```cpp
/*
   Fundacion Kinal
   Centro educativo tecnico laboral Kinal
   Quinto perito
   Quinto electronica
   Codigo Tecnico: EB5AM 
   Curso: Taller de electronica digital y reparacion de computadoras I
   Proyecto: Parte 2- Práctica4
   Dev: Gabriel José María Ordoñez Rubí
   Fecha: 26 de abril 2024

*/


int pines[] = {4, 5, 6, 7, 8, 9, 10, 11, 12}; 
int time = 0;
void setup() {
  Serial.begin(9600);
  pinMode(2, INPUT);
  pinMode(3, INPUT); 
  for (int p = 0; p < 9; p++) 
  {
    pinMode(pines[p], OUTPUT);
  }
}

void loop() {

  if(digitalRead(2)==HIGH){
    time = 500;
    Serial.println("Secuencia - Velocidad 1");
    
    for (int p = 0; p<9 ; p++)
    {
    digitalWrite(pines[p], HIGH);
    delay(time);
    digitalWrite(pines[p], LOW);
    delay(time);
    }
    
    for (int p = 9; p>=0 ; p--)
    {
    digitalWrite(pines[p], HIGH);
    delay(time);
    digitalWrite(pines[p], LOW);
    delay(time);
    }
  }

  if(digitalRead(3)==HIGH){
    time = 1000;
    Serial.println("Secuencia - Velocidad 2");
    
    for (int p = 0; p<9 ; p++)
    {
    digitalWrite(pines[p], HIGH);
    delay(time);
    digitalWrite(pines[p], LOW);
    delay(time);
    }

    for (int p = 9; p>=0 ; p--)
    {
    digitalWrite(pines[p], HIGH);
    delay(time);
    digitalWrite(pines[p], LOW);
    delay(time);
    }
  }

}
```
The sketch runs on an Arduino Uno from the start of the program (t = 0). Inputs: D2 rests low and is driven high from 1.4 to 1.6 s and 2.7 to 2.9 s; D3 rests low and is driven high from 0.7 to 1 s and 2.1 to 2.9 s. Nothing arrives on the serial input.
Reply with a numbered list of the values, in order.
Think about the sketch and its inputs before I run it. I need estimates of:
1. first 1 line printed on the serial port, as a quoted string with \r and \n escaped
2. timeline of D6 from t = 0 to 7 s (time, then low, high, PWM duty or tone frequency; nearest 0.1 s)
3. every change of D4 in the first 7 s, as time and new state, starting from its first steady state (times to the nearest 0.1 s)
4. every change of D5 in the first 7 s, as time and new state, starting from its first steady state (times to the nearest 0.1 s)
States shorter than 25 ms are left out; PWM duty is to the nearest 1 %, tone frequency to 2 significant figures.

1. "Secuencia - Velocidad 2\r\n"
2. 0 s low; 4.7 s high; 5.7 s low
3. 0 s low; 0.7 s high; 1.7 s low
4. 0 s low; 2.7 s high; 3.7 s low
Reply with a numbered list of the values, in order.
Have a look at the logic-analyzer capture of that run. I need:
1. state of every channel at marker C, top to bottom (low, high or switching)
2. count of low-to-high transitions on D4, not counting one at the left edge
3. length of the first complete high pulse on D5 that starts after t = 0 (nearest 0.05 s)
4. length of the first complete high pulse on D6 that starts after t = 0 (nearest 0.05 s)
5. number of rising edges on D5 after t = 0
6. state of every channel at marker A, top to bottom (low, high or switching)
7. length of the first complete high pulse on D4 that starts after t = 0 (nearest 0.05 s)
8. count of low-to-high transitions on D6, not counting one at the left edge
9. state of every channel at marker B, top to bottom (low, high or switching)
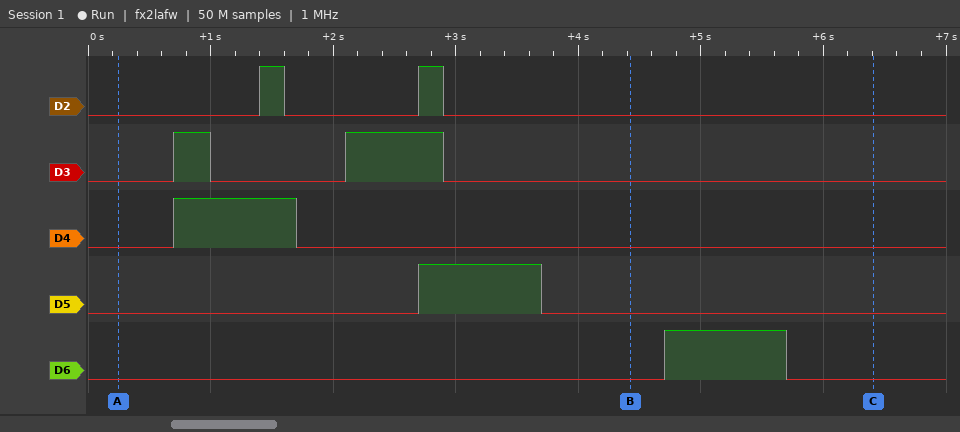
1. D2 low, D3 low, D4 low, D5 low, D6 low
2. 1
3. 1.00 s
4. 1.00 s
5. 1
6. D2 low, D3 low, D4 low, D5 low, D6 low
7. 1.00 s
8. 1
9. D2 low, D3 low, D4 low, D5 low, D6 low
